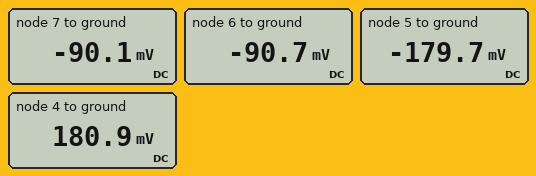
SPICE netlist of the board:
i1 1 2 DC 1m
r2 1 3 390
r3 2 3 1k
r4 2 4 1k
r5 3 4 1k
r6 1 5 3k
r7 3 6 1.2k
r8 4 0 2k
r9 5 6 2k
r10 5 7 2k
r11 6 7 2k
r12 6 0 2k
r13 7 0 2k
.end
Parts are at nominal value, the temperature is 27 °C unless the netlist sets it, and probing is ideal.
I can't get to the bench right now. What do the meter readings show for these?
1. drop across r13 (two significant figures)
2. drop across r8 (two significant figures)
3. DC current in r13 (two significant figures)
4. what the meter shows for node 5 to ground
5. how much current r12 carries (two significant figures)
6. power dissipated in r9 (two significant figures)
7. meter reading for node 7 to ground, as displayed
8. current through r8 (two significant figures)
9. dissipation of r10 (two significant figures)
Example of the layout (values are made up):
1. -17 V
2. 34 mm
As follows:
1. 90 mV
2. 180 mV
3. 45 µA
4. -179.7 mV
5. 45 µA
6. 4.0 µW
7. -90.1 mV
8. 90 µA
9. 4.0 µW
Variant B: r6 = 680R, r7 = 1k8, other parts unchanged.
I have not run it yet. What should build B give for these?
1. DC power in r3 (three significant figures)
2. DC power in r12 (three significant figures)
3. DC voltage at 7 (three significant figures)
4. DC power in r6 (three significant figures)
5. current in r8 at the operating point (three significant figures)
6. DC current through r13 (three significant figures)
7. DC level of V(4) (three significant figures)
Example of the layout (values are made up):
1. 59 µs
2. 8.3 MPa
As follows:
1. 396 µW
2. 5.28 µW
3. -122 mV
4. 15.4 µW
5. 112 µA
6. 60.9 µA
7. 225 mV
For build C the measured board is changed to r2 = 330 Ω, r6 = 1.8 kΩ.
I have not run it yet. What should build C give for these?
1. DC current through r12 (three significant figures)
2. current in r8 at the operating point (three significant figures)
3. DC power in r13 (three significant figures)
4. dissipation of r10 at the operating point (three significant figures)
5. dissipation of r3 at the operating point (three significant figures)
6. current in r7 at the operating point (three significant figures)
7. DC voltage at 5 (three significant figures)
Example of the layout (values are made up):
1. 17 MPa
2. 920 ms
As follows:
1. 46.0 µA
2. 94.0 µA
3. 4.60 µW
4. 4.99 µW
5. 404 µW
6. 7.81 µA
7. -196 mV
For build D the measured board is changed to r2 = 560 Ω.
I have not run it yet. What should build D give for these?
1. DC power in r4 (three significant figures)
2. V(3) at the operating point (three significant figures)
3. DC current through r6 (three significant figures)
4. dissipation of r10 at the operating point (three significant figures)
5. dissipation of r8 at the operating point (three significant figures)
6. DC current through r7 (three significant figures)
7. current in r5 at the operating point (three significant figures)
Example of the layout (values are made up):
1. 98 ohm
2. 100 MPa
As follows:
1. 134 µW
2. -71.3 mV
3. 117 µA
4. 6.30 µW
5. 19.3 µW
6. 18.6 µA
7. 268 µA
